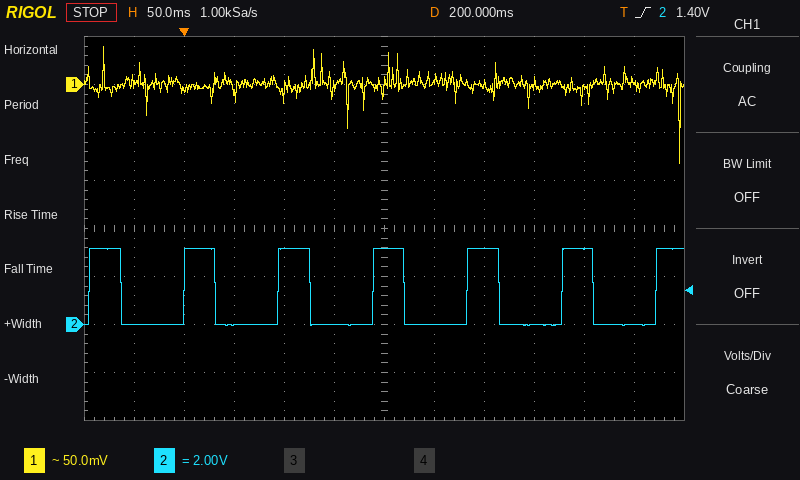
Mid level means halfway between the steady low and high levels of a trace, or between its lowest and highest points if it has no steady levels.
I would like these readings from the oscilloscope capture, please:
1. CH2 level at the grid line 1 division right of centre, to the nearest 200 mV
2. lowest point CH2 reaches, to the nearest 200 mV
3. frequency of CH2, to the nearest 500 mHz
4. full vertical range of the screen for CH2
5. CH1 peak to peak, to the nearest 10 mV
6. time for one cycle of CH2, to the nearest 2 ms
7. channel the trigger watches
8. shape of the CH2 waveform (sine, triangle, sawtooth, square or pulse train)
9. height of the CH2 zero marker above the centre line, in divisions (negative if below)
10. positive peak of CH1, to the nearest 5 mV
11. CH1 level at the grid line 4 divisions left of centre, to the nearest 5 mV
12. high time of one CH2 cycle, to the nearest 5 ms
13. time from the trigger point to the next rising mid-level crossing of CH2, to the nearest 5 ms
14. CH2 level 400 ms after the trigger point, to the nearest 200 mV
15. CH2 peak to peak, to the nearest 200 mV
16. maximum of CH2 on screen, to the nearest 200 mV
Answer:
0.0 V
0.0 V
10.5 Hz
16 V
120 mV
94 ms
CH2
pulse train
-2.0 div
40 mV
-5 mV
30 ms
95 ms
3.2 V
3.2 V
3.2 V
